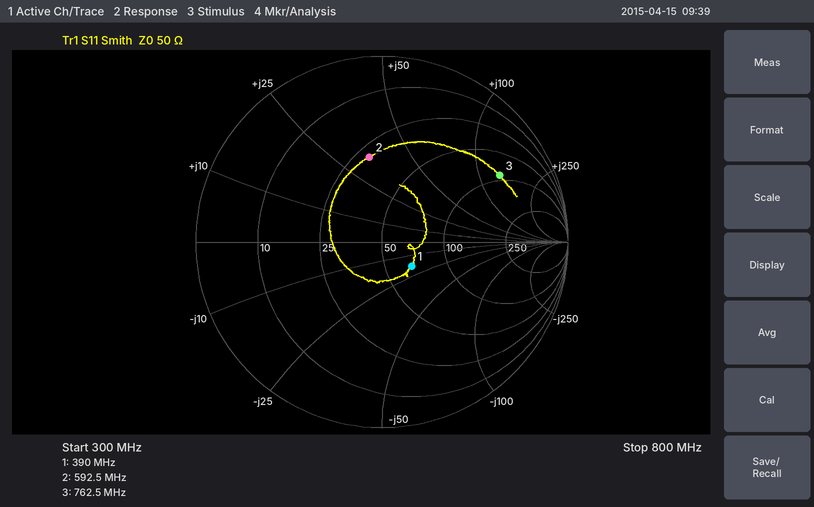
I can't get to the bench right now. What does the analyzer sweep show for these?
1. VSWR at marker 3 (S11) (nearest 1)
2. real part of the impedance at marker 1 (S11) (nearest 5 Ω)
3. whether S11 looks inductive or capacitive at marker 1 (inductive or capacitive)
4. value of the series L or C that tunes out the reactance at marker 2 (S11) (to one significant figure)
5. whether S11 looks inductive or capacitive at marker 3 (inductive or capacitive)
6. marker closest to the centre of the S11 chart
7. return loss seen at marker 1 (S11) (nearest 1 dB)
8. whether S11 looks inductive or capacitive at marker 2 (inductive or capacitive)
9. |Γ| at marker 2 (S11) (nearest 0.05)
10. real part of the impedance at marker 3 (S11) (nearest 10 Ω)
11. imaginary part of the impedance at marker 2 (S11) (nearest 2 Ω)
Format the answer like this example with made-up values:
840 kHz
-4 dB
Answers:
6
65 Ω
capacitive
8 pF
inductive
marker 1
14 dB
inductive
0.45
90 Ω
+34 Ω
